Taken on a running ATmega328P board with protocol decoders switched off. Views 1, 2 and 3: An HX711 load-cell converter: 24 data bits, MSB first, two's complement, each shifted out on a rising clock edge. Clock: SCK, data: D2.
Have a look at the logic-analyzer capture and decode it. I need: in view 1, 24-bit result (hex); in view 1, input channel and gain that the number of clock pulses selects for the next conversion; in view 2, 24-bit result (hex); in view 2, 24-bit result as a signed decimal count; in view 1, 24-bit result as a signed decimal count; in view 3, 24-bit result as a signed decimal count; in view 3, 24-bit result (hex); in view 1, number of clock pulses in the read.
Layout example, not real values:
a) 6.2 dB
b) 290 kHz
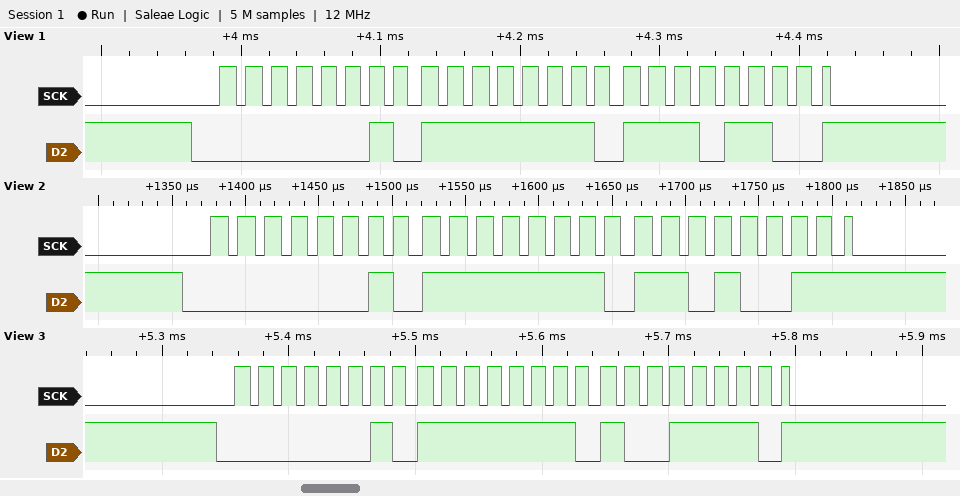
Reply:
a) 0x02FEEC
b) channel A, gain 128
c) 0x02FED3
d) 196307
e) 196332
f) 196254
g) 0x02FE9E
h) 25
